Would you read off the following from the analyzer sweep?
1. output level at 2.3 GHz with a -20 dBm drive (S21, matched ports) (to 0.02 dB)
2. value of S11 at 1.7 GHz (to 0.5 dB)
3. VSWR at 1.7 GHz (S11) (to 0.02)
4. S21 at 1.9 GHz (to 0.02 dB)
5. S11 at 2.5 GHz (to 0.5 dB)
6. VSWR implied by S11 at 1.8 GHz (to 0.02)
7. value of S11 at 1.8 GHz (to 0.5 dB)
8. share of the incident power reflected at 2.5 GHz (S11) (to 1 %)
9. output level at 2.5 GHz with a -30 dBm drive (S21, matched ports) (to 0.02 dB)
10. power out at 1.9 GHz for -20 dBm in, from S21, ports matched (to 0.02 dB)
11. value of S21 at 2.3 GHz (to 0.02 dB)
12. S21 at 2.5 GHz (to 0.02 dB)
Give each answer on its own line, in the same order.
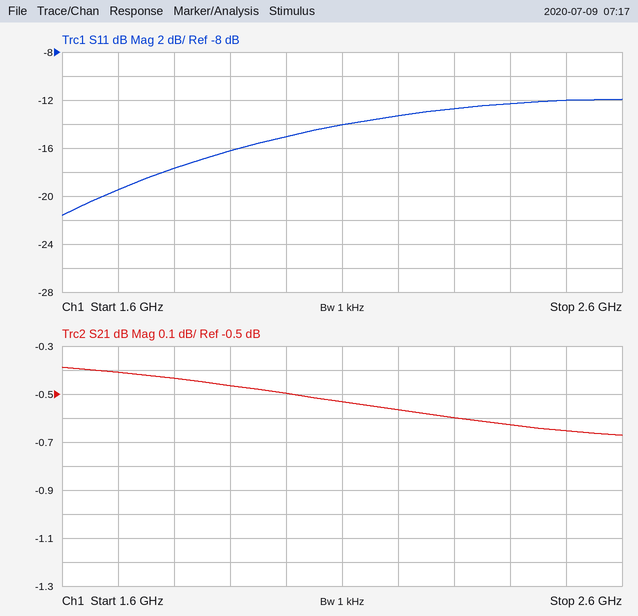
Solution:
-20.60 dBm
-19.5 dB
1.24
-0.46 dB
-12.0 dB
1.30
-17.5 dB
6 %
-30.66 dBm
-20.46 dBm
-0.60 dB
-0.66 dB
